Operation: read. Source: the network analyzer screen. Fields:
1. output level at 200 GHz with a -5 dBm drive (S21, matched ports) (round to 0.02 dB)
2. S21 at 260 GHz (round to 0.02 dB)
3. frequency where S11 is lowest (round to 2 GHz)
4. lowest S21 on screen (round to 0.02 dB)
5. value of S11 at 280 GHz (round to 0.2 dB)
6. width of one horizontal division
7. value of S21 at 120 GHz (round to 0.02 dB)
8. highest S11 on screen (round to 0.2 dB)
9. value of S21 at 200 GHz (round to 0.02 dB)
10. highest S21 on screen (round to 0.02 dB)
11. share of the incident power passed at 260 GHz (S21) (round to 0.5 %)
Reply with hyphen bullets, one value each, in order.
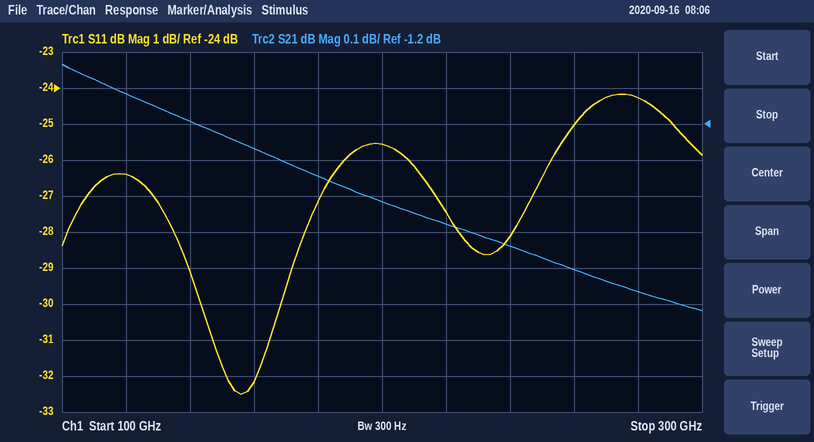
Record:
- -6.42 dBm
- -1.60 dB
- 156 GHz
- -1.72 dB
- -24.2 dB
- 20 GHz
- -1.12 dB
- -24.2 dB
- -1.42 dB
- -1.04 dB
- 69.0 %
